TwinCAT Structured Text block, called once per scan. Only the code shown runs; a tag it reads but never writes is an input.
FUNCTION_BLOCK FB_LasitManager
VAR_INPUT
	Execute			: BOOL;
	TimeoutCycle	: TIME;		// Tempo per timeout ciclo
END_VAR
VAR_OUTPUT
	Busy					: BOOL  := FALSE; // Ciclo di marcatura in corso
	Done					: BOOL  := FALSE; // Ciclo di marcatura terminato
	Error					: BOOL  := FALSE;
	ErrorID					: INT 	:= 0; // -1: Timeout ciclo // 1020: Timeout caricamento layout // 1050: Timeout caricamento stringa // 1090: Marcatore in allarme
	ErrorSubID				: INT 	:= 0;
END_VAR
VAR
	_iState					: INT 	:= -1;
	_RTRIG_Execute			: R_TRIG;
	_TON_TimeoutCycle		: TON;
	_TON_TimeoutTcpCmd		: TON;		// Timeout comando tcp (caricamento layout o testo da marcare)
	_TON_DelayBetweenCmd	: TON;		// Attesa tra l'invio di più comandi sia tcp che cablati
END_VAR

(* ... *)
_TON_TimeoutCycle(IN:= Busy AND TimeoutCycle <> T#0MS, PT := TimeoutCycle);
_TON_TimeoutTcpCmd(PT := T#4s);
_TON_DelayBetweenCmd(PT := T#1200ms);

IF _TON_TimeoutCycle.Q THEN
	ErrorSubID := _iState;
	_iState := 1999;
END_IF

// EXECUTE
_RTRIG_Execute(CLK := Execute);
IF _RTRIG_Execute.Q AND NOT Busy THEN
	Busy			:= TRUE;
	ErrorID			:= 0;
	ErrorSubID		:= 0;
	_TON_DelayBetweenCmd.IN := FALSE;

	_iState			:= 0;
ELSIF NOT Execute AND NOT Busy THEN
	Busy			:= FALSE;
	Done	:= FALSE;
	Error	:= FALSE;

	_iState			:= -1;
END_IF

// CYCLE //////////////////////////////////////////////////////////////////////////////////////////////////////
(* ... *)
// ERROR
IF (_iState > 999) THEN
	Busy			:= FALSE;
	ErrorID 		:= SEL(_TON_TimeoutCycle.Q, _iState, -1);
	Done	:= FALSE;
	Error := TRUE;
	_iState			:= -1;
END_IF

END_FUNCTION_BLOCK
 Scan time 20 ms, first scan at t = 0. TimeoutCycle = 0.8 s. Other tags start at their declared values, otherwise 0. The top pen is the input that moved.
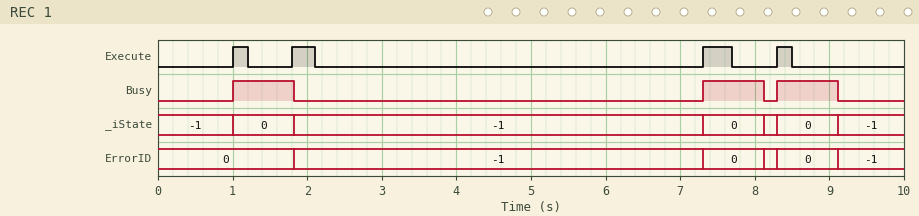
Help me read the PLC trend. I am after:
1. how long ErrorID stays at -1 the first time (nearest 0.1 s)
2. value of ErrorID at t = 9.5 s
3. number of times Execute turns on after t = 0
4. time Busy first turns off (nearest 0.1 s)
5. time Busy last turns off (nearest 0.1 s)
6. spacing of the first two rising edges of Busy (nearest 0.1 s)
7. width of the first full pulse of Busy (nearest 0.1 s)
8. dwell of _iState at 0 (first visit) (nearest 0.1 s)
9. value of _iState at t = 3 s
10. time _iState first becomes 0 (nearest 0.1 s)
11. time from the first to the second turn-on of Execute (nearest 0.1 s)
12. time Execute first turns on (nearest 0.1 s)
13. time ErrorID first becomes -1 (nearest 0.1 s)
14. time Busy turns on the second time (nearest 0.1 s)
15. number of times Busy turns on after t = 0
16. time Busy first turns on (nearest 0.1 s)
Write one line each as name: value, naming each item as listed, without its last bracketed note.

how long ErrorID stays at -1 the first time: 5.5 s
value of ErrorID at t = 9.5 s: -1
number of times Execute turns on after t = 0: 4
time Busy first turns off: 1.8 s
time Busy last turns off: 9.1 s
spacing of the first two rising edges of Busy: 6.3 s
width of the first full pulse of Busy: 0.8 s
dwell of _iState at 0 (first visit): 0.8 s
value of _iState at t = 3 s: -1
time _iState first becomes 0: 1.0 s
time from the first to the second turn-on of Execute: 0.8 s
time Execute first turns on: 1.0 s
time ErrorID first becomes -1: 1.8 s
time Busy turns on the second time: 7.3 s
number of times Busy turns on after t = 0: 3
time Busy first turns on: 1.0 s
